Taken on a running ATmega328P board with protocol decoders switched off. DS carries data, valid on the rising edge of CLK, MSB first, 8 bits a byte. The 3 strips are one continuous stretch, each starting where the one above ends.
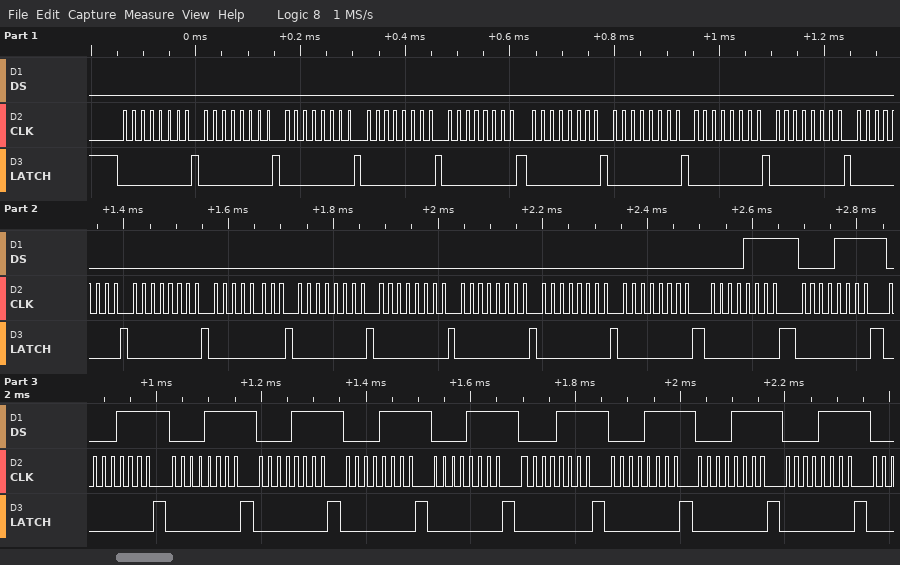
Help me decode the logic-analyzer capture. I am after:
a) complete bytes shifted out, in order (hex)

0x00 0x00 0x00 0x00 0x00 0x00 0x00 0x00 0x00 0x00 0x00 0x00 0x00 0x00 0x00 0x00 0x00 0x0F 0x0F 0x0F 0x0F 0x0F 0x0F 0x0F 0x0F 0x0F 0x0F 0x0F
